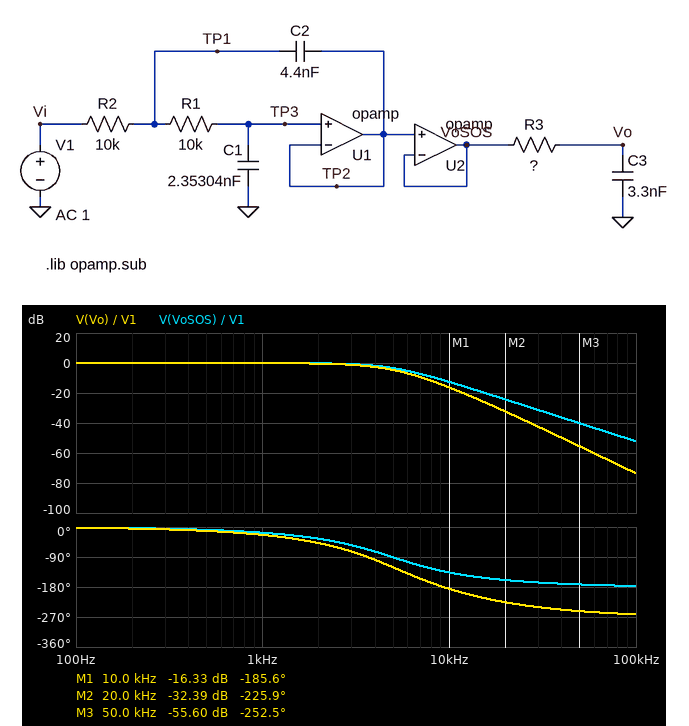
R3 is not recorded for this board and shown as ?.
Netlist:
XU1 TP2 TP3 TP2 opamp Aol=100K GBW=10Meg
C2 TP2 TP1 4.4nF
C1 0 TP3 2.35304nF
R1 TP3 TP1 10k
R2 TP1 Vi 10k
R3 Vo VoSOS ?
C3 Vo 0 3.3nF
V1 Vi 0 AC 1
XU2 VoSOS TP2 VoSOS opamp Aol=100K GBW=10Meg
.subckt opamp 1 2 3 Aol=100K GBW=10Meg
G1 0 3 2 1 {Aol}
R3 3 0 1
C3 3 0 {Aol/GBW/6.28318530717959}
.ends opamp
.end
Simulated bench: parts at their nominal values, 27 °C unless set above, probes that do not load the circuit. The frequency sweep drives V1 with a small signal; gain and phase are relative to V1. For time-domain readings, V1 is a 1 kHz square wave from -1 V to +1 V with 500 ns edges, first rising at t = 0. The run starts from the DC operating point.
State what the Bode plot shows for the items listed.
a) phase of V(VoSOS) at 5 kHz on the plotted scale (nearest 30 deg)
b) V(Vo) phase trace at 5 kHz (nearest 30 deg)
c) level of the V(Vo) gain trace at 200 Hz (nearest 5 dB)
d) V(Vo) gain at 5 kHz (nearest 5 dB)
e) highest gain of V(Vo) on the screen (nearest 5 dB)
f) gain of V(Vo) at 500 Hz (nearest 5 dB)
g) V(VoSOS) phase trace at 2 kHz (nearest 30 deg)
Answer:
-90 deg
-120 deg
0 dB
-5 dB
0 dB
0 dB
-30 deg
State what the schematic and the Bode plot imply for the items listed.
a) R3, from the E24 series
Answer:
5.6 kΩ
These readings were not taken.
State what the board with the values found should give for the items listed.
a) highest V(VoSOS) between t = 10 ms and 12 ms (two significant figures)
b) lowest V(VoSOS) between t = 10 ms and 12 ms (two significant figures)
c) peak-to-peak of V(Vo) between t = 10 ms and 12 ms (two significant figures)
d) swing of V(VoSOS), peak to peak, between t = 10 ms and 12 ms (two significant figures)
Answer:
1.1 V
-1.1 V
2.1 V
2.1 V
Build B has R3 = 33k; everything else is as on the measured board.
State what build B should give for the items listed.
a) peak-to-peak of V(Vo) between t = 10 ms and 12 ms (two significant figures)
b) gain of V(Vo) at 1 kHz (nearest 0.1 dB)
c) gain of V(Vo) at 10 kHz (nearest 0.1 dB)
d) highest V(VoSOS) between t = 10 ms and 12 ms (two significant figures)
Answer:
1.9 V
-1.7 dB
-29.4 dB
1.1 V
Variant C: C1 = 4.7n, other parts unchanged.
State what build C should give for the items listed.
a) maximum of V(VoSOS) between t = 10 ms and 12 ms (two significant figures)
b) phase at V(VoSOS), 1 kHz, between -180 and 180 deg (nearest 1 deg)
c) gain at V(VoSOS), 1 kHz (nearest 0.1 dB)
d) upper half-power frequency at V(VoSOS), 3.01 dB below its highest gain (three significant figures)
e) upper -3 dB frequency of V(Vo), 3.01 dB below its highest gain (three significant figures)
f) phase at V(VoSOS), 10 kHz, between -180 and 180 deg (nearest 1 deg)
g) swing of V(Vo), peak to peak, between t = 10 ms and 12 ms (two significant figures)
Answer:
1.0 V
-33 deg
-0.8 dB
2.15 kHz
2.05 kHz
-141 deg
2.0 V
